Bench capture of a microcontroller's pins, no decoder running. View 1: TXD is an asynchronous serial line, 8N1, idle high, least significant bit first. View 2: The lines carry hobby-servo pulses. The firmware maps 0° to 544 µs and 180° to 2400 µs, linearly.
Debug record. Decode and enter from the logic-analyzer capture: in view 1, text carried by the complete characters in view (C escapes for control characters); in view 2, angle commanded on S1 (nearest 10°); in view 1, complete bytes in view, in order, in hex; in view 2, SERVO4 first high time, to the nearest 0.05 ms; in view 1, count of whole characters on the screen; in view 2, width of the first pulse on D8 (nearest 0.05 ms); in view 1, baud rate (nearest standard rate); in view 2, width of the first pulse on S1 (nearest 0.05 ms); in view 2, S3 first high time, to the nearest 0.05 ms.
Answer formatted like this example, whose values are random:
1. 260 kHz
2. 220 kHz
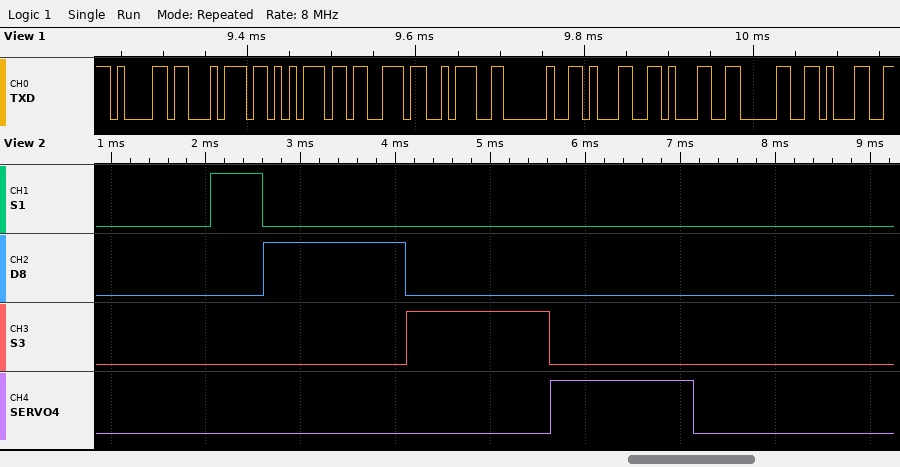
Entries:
1. "atus: 1101"
2. 0°
3. 61 74 75 73 3A 20 31 31 30 31
4. 1.50 ms
5. 10
6. 1.50 ms
7. 115200 baud
8. 0.55 ms
9. 1.50 ms
